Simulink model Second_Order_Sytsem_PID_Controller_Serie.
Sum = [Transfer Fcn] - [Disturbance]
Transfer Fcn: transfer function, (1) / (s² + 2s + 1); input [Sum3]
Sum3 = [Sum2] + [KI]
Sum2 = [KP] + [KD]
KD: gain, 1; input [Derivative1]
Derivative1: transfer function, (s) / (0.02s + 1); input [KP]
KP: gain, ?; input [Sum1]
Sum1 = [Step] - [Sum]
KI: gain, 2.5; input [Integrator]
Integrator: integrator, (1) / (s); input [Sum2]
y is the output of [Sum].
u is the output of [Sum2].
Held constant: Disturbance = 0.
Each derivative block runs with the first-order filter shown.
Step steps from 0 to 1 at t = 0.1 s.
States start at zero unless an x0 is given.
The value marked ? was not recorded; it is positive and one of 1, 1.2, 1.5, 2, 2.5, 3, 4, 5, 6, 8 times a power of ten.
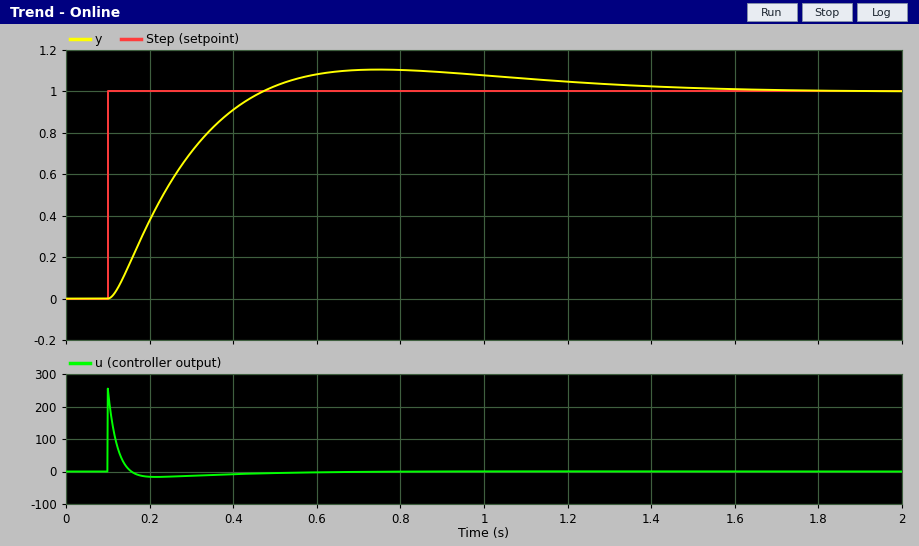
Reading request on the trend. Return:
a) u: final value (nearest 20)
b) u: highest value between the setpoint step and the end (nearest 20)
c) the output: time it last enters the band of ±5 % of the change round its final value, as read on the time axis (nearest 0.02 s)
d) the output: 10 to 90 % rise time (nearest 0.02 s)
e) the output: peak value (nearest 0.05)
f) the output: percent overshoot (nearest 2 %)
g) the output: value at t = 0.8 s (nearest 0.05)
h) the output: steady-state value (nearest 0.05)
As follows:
0
260
1.18 s
0.26 s
1.10
10 %
1.10
1.00
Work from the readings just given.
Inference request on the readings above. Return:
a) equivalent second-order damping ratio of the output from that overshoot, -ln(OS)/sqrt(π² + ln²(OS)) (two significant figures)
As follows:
0.59
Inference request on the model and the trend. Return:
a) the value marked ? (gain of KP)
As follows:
5
